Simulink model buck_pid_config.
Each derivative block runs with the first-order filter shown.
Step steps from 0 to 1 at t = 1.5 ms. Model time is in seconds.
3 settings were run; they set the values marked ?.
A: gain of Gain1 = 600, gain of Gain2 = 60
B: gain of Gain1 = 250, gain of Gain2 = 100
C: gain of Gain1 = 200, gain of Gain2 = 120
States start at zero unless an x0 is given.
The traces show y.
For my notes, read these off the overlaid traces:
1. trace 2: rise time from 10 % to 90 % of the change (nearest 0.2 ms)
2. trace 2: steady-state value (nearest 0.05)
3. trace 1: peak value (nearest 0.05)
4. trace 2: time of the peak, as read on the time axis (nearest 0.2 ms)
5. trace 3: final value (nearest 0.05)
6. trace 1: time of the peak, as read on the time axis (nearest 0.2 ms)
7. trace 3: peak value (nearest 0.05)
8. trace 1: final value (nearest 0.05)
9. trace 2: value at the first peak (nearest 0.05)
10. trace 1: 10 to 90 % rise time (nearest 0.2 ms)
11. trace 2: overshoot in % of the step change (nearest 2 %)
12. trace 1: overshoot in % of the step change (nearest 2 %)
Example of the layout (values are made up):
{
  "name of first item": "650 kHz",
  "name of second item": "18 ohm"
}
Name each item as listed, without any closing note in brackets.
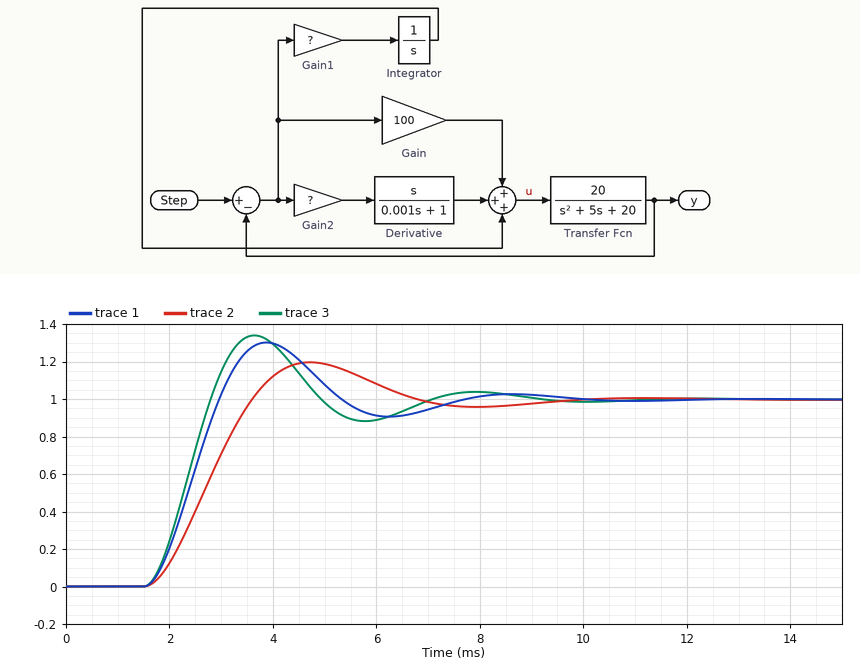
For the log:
{
  "trace 2: rise time from 10 % to 90 % of the change": "1.4 ms",
  "trace 2: steady-state value": "1.00",
  "trace 1: peak value": "1.30",
  "trace 2: time of the peak, as read on the time axis": "4.8 ms",
  "trace 3: final value": "1.00",
  "trace 1: time of the peak, as read on the time axis": "3.8 ms",
  "trace 3: peak value": "1.35",
  "trace 1: final value": "1.00",
  "trace 2: value at the first peak": "1.20",
  "trace 1: 10 to 90 % rise time": "1.0 ms",
  "trace 2: overshoot in % of the step change": "20 %",
  "trace 1: overshoot in % of the step change": "30 %"
}
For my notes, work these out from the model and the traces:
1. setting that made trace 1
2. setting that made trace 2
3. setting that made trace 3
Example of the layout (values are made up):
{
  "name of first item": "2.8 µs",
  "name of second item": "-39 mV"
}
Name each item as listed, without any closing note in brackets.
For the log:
{
  "setting that made trace 1": "B",
  "setting that made trace 2": "A",
  "setting that made trace 3": "C"
}
